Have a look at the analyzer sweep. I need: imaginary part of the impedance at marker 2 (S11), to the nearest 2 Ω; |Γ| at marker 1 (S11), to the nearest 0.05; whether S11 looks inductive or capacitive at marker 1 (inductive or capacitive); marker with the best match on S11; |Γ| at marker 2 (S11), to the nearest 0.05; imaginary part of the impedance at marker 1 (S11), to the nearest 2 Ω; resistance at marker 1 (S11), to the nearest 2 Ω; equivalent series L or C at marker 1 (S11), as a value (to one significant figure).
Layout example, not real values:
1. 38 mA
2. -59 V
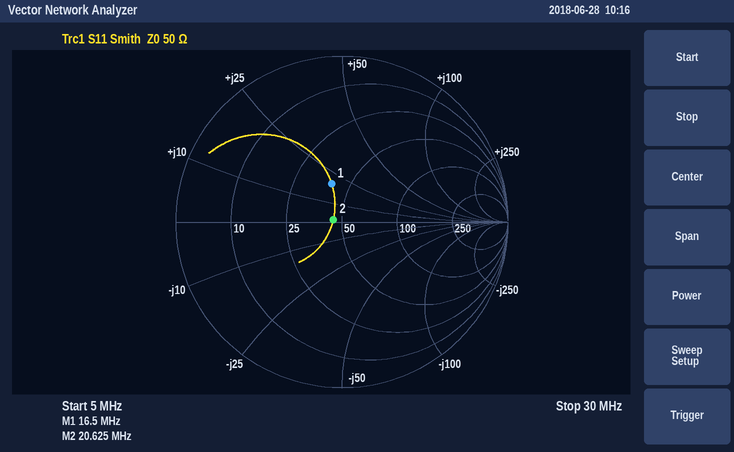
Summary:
1. +2 Ω
2. 0.25
3. inductive
4. marker 2
5. 0.05
6. +20 Ω
7. 40 Ω
8. 200 nH
